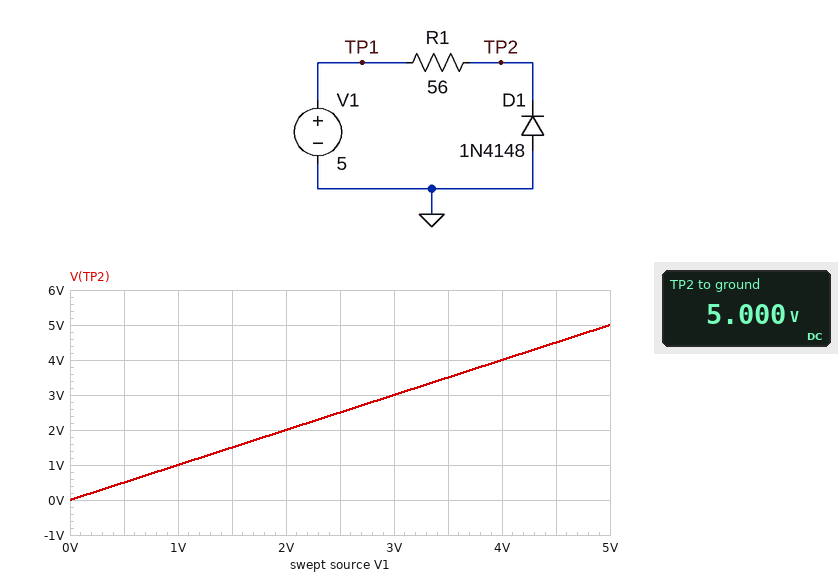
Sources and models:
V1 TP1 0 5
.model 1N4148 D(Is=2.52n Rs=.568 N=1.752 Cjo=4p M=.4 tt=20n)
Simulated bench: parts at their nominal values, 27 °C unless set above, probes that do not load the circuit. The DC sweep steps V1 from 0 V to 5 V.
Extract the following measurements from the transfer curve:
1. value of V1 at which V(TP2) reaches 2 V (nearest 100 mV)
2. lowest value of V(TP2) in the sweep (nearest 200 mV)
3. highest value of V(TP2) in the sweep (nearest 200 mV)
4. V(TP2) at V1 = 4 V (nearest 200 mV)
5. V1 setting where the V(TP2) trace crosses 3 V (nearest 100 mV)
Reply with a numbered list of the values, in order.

1. 2.0 V
2. 0 V
3. 5.0 V
4. 4.0 V
5. 3.0 V
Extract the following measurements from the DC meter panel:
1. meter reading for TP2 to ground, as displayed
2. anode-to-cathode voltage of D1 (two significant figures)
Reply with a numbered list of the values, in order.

1. 5.000 V
2. -5.0 V
